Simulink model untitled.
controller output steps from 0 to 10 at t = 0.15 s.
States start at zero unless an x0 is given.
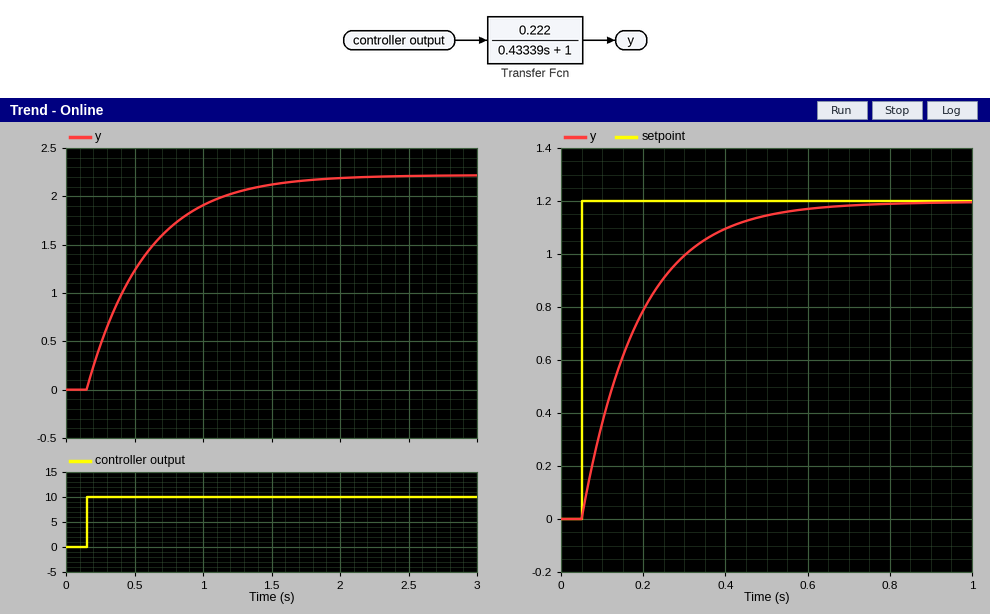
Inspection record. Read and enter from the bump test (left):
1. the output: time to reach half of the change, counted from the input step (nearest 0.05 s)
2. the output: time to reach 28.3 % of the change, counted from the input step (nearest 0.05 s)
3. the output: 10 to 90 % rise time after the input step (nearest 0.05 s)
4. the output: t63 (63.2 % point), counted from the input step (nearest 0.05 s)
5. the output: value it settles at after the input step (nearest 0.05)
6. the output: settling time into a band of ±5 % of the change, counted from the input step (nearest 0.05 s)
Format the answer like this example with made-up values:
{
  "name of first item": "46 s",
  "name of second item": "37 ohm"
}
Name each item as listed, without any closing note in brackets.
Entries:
{
  "the output: time to reach half of the change, counted from the input step": "0.30 s",
  "the output: time to reach 28.3 % of the change, counted from the input step": "0.15 s",
  "the output: 10 to 90 % rise time after the input step": "0.95 s",
  "the output: t63 (63.2 % point), counted from the input step": "0.45 s",
  "the output: value it settles at after the input step": "2.20",
  "the output: settling time into a band of ±5 % of the change, counted from the input step": "1.30 s"
}
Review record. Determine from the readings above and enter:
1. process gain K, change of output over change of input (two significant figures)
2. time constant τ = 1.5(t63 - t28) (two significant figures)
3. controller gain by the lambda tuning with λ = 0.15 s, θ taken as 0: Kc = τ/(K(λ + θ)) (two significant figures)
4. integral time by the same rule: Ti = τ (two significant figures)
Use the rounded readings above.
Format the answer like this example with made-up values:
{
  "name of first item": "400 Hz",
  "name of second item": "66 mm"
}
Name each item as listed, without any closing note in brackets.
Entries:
{
  "process gain K, change of output over change of input": "0.22",
  "time constant τ = 1.5(t63 - t28)": "0.45 s",
  "controller gain by the lambda tuning with λ = 0.15 s, θ taken as 0: Kc = τ/(K(λ + θ))": "14",
  "integral time by the same rule: Ti = τ": "0.45 s"
}
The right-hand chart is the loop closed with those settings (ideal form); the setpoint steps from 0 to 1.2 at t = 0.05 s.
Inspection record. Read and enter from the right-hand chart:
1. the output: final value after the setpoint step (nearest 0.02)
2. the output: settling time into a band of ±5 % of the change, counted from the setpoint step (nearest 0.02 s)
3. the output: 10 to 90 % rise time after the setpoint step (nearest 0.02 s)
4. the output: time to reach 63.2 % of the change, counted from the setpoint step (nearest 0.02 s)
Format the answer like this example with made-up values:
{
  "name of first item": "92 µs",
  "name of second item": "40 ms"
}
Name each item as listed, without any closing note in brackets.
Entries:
{
  "the output: final value after the setpoint step": "1.20",
  "the output: settling time into a band of ±5 % of the change, counted from the setpoint step": "0.44 s",
  "the output: 10 to 90 % rise time after the setpoint step": "0.32 s",
  "the output: time to reach 63.2 % of the change, counted from the setpoint step": "0.14 s"
}
